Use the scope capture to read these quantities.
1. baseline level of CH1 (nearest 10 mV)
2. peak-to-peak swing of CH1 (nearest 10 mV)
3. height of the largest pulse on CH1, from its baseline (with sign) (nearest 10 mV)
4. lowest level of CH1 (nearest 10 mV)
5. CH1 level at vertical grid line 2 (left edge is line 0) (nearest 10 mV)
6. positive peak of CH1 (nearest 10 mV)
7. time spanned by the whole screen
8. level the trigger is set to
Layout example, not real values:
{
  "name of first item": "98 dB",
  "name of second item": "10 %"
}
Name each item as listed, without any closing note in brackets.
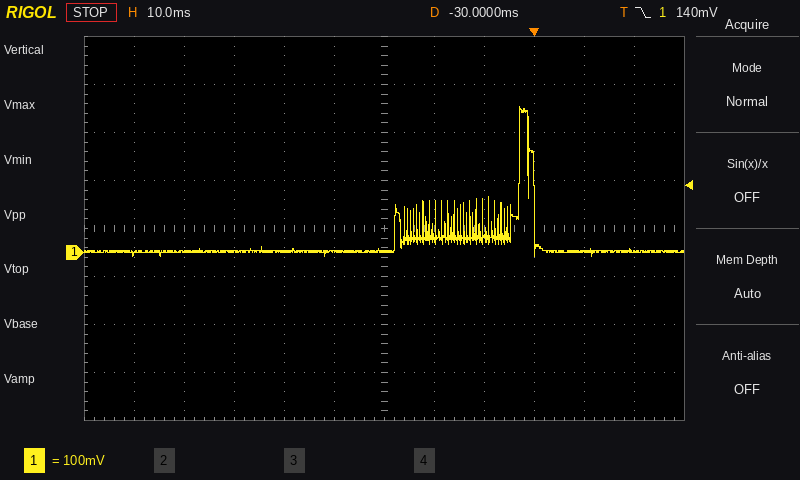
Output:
{
  "baseline level of CH1": "0 mV",
  "peak-to-peak swing of CH1": "310 mV",
  "height of the largest pulse on CH1, from its baseline (with sign)": "+300 mV",
  "lowest level of CH1": "-10 mV",
  "CH1 level at vertical grid line 2 (left edge is line 0)": "0 mV",
  "positive peak of CH1": "300 mV",
  "time spanned by the whole screen": "120 ms",
  "level the trigger is set to": "140 mV"
}
